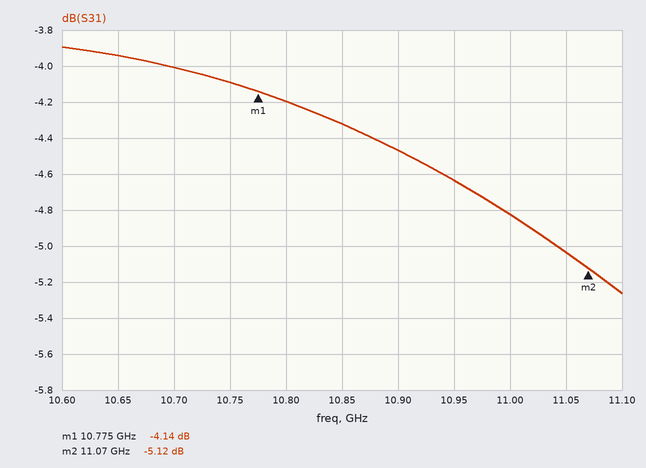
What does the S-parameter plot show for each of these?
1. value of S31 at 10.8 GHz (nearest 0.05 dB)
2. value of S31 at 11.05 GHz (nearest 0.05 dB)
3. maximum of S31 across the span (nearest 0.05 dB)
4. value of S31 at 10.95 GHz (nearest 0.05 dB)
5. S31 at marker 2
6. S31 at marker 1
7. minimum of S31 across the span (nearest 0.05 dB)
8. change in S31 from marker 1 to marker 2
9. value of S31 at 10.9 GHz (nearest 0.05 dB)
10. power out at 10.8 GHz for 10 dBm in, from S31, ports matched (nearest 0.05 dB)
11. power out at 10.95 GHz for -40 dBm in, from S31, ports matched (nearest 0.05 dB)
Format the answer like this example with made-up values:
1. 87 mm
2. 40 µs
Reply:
1. -4.20 dB
2. -5.05 dB
3. -3.90 dB
4. -4.65 dB
5. -5.12 dB
6. -4.14 dB
7. -5.25 dB
8. -0.98 dB
9. -4.45 dB
10. 5.80 dBm
11. -44.65 dBm
